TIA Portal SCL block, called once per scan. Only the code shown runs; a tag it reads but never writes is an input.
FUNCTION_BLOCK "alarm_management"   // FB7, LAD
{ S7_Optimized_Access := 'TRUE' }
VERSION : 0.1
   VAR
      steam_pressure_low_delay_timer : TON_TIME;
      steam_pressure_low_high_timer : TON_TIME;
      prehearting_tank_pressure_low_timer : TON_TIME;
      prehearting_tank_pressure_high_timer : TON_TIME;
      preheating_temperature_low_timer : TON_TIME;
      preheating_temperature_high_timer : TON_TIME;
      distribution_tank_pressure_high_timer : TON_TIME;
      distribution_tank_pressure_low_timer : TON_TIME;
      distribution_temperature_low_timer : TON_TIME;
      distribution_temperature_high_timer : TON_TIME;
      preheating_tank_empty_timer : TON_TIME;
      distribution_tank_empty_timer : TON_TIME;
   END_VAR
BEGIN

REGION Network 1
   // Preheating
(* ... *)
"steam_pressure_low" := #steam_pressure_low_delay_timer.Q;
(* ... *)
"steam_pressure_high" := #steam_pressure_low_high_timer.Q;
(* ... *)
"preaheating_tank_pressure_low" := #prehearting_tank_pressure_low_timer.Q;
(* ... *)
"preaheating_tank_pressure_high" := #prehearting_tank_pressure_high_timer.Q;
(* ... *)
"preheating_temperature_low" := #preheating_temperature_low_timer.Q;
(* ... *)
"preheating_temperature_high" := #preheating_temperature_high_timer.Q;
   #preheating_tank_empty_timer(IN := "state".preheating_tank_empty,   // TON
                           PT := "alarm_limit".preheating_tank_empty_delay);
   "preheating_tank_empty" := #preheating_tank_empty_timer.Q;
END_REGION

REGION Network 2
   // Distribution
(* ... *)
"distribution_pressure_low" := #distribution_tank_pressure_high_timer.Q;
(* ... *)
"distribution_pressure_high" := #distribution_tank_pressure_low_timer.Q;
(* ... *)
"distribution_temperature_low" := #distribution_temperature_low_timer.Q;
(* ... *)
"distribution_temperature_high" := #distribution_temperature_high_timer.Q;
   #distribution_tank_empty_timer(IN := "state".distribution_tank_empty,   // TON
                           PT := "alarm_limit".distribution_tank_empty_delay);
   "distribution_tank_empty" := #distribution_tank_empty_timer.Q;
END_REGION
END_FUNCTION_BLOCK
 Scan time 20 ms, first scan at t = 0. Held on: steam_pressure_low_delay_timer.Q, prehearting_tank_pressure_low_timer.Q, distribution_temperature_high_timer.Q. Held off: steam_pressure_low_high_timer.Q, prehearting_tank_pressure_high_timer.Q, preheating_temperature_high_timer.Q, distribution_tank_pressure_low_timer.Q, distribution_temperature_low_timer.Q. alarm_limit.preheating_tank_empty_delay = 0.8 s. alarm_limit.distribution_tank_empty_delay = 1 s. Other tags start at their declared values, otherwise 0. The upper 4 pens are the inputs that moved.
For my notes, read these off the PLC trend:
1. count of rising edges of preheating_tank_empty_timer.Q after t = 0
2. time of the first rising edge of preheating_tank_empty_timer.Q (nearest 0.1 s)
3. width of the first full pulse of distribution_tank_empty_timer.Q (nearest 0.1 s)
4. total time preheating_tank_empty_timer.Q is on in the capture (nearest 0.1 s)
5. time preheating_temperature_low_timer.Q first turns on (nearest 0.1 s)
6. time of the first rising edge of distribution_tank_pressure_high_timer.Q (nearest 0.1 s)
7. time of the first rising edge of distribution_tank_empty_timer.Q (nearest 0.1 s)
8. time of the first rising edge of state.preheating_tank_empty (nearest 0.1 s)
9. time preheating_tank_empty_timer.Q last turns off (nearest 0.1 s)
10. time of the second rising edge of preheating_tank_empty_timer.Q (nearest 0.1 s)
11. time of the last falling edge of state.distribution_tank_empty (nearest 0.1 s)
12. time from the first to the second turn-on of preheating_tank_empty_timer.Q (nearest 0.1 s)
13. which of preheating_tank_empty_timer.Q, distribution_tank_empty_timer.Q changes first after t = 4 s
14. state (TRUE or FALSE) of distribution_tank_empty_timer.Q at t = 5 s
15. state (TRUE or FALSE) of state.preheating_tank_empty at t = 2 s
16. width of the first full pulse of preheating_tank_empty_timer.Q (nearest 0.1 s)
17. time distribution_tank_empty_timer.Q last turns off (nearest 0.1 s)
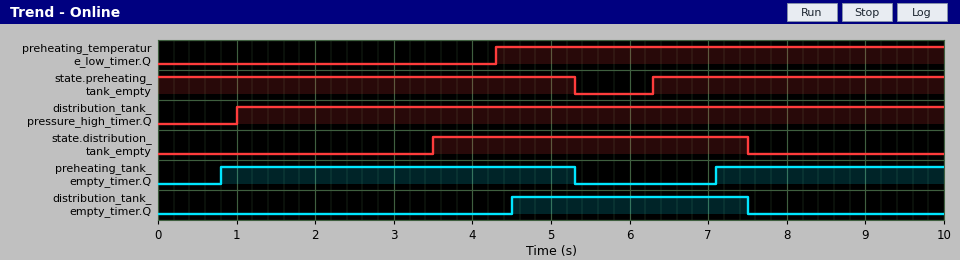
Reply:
2
0.8 s
3.0 s
7.4 s
4.3 s
1.0 s
4.5 s
6.3 s
5.3 s
7.1 s
7.5 s
6.3 s
distribution_tank_empty_timer.Q
TRUE
TRUE
4.5 s
7.5 s
